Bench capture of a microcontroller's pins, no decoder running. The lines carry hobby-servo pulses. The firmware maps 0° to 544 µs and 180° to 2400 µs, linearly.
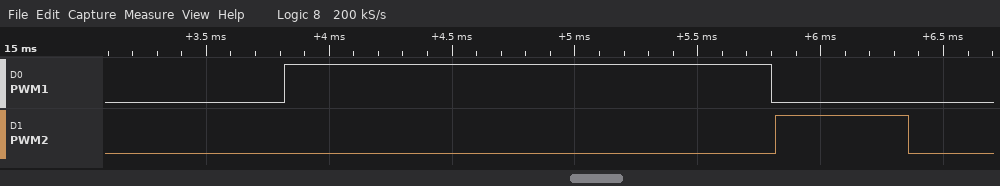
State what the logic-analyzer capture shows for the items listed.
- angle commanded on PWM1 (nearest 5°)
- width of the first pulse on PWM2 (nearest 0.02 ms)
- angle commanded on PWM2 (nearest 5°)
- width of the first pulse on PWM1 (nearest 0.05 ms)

140°
0.54 ms
0°
2.00 ms
